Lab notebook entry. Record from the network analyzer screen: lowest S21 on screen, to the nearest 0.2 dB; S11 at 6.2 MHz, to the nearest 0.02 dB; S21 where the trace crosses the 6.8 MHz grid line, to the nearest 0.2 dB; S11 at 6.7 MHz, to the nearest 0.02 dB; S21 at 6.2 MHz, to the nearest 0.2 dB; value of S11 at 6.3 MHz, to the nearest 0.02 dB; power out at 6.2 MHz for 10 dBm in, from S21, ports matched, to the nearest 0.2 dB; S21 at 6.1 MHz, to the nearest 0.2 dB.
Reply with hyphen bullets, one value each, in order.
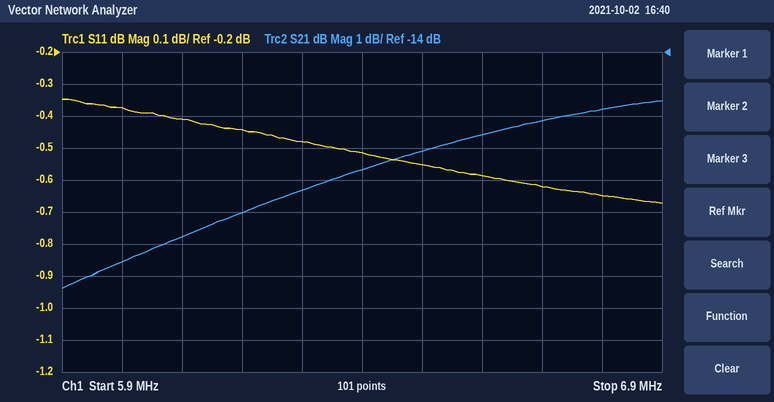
- -21.4 dB
- -0.44 dB
- -15.8 dB
- -0.62 dB
- -19.0 dB
- -0.48 dB
- -9.0 dBm
- -19.8 dB
